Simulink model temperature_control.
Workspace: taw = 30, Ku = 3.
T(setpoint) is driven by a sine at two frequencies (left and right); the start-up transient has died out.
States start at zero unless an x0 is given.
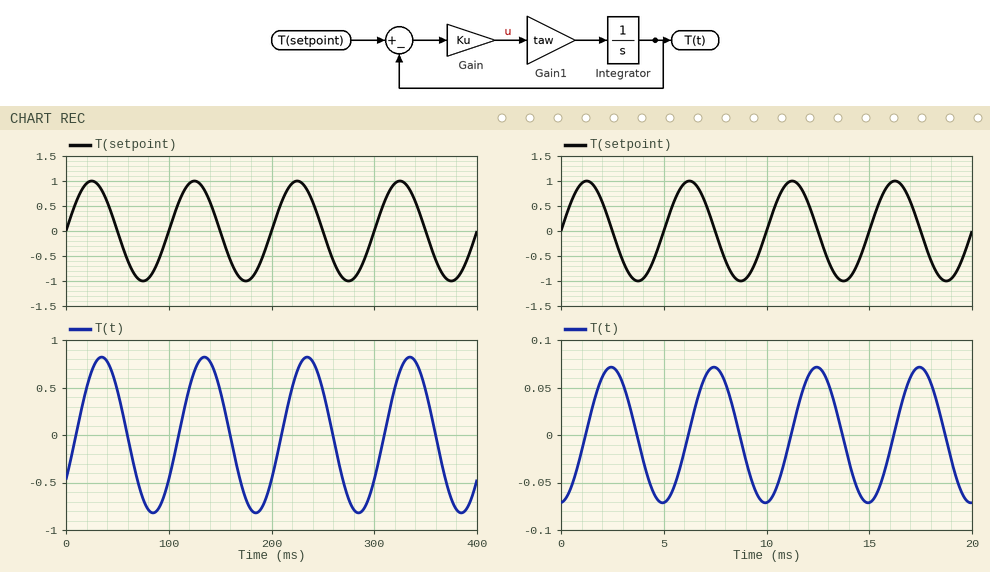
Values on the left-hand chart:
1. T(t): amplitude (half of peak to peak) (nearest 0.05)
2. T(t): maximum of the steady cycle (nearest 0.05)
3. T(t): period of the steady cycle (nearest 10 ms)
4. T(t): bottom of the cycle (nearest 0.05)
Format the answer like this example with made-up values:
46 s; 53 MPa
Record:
0.80; 0.80; 100 ms; -0.80
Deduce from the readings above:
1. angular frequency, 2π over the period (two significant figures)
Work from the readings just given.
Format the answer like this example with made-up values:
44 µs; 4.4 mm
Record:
0.063 rad/ms
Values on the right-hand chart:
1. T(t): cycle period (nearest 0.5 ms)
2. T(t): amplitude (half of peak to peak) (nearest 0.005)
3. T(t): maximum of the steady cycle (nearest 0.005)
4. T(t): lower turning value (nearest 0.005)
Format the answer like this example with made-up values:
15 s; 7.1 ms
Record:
5.0 ms; 0.070; 0.070; -0.070
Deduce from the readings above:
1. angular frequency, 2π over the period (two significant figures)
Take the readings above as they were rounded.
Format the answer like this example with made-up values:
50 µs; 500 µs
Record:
1.3 rad/ms
